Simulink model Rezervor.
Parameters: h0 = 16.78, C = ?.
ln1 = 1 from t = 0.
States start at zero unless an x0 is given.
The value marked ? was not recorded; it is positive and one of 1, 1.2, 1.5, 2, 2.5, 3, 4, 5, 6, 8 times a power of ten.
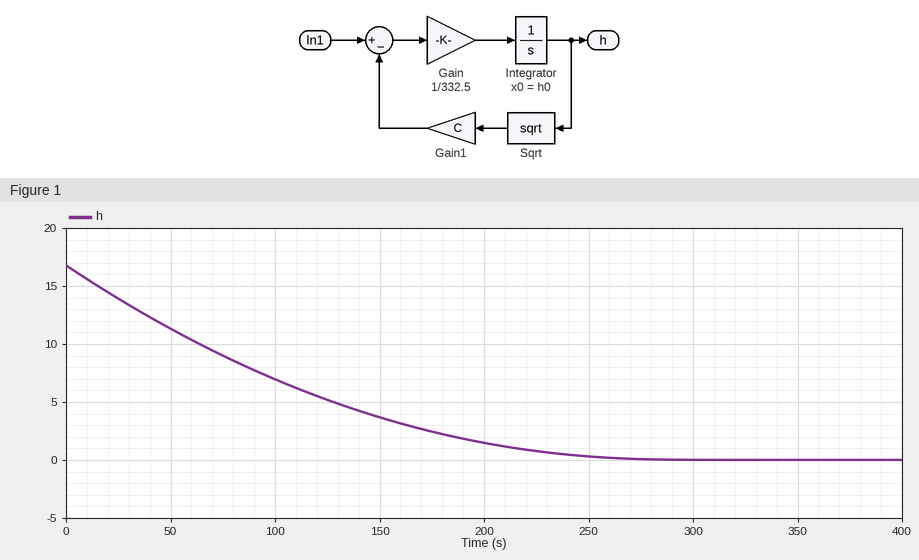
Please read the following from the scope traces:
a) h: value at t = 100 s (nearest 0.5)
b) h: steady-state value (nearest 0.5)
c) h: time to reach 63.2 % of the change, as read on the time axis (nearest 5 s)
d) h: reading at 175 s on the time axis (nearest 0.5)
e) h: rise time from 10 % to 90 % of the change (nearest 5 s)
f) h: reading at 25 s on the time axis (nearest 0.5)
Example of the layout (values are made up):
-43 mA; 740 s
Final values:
7.0; 0.0; 110 s; 2.5; 180 s; 14.0
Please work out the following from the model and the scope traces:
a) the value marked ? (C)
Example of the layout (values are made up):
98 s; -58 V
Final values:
10
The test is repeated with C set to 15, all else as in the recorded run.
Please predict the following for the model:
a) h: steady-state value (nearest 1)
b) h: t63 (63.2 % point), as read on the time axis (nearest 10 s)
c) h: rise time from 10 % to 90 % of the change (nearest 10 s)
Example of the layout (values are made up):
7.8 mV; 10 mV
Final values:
0; 70 s; 120 s
